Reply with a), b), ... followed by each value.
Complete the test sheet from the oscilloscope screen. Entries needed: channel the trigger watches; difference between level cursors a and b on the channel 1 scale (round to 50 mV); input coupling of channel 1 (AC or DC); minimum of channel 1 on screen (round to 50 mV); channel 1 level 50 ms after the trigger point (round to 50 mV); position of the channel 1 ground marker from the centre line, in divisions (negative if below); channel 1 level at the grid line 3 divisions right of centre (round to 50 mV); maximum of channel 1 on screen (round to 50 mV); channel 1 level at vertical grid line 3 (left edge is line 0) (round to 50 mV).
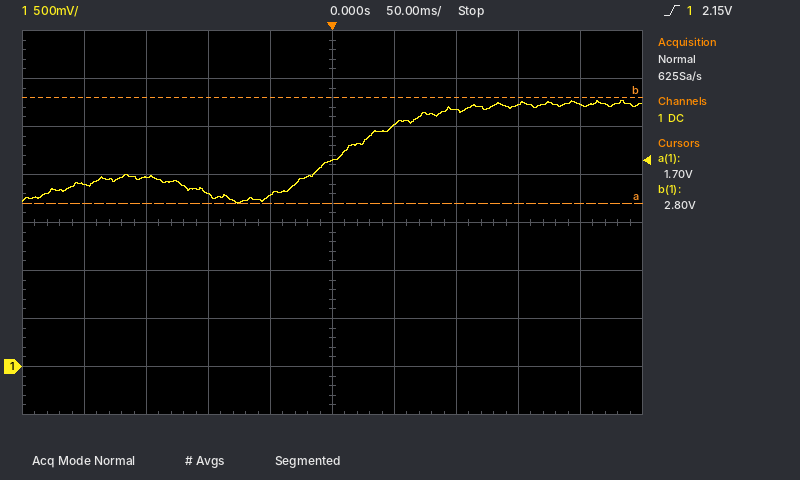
a) channel 1
b) 1.10 V
c) DC
d) 1.70 V
e) 2.50 V
f) -3.0 div
g) 2.75 V
h) 2.75 V
i) 1.80 V
